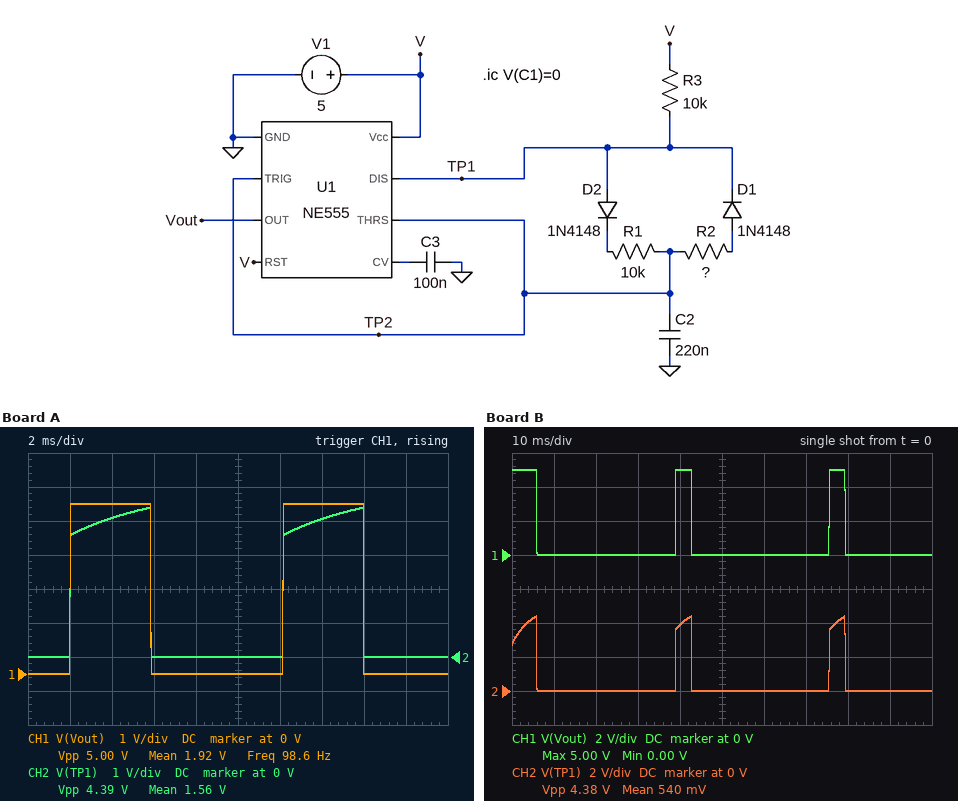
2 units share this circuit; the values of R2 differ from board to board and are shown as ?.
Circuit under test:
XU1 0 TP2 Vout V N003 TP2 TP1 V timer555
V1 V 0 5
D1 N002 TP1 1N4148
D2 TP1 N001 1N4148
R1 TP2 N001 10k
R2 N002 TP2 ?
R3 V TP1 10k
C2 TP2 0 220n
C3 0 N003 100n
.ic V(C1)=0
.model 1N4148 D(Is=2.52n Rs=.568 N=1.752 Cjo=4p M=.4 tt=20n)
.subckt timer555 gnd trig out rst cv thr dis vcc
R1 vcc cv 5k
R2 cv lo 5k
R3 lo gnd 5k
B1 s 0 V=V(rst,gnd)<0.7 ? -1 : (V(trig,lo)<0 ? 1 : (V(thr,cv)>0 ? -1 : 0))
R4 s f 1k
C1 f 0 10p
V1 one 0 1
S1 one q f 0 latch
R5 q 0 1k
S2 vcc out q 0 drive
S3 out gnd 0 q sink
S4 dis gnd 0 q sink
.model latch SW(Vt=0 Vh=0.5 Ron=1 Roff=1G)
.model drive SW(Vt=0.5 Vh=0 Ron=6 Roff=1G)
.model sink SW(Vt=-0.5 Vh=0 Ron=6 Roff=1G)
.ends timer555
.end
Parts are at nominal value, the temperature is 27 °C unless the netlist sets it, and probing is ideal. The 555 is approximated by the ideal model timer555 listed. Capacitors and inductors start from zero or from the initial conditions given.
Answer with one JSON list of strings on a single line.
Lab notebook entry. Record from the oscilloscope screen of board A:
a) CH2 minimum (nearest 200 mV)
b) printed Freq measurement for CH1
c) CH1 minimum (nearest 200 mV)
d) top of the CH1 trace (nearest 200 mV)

["0 V", "98.6 Hz", "0 V", "5.0 V"]
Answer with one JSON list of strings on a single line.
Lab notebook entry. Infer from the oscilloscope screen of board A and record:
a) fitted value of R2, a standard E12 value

["33 kΩ"]
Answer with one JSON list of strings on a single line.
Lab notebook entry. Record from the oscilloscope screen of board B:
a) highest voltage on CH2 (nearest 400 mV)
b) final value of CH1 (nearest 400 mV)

["4.4 V", "0 V"]
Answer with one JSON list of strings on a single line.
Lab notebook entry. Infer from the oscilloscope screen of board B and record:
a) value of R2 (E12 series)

["180 kΩ"]
